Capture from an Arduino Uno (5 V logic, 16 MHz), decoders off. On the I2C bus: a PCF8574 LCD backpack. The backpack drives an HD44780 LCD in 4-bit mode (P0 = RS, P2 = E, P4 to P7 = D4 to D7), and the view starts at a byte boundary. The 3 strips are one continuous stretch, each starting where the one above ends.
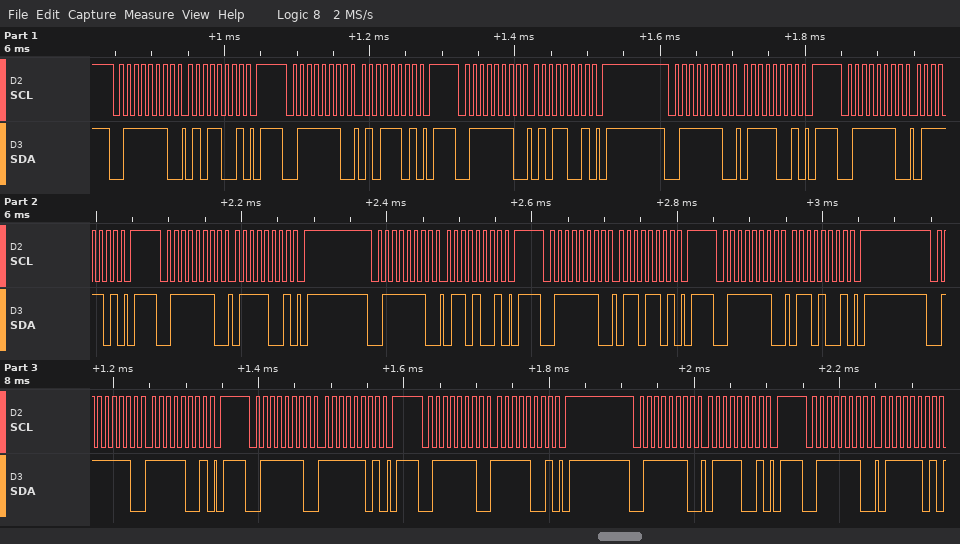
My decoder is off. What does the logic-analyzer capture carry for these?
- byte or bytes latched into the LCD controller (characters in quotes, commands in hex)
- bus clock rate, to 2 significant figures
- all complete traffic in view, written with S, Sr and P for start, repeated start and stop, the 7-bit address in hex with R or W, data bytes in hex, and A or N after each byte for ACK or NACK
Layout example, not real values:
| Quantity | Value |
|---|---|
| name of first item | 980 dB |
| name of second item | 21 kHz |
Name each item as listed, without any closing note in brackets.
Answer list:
| Quantity | Value |
|---|---|
| byte or bytes latched into the LCD controller | 'W' 'o' |
| bus clock rate, to 2 significant figures | 100 kHz |
| all complete traffic in view, written with S, Sr and P for start, repeated start and stop, the 7-bit address in hex with R or W, data bytes in hex, and A or N after each byte for ACK or NACK | S 3FW A 59 A P S 3FW A 5D A P S 3FW A 59 A P S 3FW A 79 A P S 3FW A 7D A P S 3FW A 79 A P S 3FW A 69 A P S 3FW A 6D A P S 3FW A 69 A P S 3FW A F9 A P S 3FW A FD A P S 3FW A F9 A P S 3FW A 79 A P S 3FW A 7D A |
